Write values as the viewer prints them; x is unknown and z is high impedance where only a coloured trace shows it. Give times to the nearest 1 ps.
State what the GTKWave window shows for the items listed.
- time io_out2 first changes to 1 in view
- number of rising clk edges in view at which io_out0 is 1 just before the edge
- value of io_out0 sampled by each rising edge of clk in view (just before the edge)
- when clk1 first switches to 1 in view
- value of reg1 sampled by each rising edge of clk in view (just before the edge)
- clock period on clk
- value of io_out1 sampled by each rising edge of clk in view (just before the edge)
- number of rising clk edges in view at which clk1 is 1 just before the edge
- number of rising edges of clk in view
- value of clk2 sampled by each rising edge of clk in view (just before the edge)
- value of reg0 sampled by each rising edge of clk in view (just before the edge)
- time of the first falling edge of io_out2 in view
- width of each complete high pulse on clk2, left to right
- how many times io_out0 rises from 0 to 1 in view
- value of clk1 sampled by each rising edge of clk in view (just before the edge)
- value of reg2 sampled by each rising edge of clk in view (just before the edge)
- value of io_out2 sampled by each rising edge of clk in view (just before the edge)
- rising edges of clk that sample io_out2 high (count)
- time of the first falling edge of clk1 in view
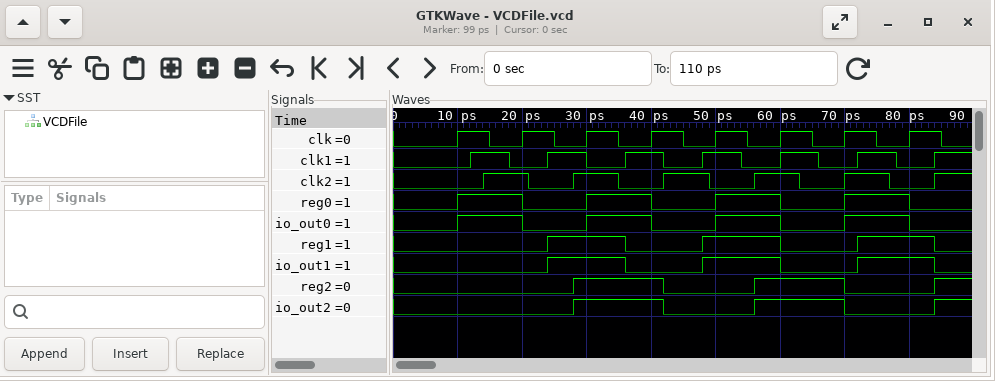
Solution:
28 ps
4
0 1 0 1 0 1 0 1
12 ps
0 0 1 0 1 1 0 1
10 ps
0 0 1 0 1 1 0 1
3
8
0 1 1 0 0 1 0 0
0 1 0 1 0 1 0 1
42 ps
7 ps, 7 ps, 7 ps, 7 ps, 7 ps
4
0 0 1 1 1 0 0 0
0 0 1 1 0 1 1 0
0 0 1 1 0 1 1 0
4
18 ps
